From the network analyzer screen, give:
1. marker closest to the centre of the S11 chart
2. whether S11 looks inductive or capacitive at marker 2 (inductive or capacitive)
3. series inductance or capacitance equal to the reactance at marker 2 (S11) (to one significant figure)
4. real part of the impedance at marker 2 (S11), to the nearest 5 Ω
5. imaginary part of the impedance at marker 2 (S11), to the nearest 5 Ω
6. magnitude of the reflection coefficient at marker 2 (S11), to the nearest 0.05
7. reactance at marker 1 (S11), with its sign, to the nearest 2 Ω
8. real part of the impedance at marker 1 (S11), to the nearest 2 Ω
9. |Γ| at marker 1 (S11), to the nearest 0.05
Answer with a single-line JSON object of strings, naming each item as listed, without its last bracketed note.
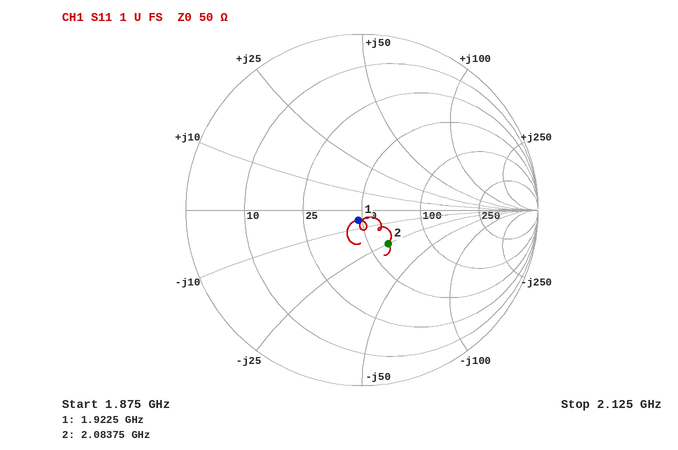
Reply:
{"marker closest to the centre of the S11 chart": "marker 1", "whether S11 looks inductive or capacitive at marker 2": "capacitive", "series inductance or capacitance equal to the reactance at marker 2 (S11)": "3 pF", "real part of the impedance at marker 2 (S11), to the nearest 5 Ω": "60 Ω", "imaginary part of the impedance at marker 2 (S11), to the nearest 5 Ω": "-25 Ω", "magnitude of the reflection coefficient at marker 2 (S11), to the nearest 0.05": "0.25", "reactance at marker 1 (S11), with its sign, to the nearest 2 Ω": "-6 Ω", "real part of the impedance at marker 1 (S11), to the nearest 2 Ω": "48 Ω", "|Γ| at marker 1 (S11), to the nearest 0.05": "0.05"}
